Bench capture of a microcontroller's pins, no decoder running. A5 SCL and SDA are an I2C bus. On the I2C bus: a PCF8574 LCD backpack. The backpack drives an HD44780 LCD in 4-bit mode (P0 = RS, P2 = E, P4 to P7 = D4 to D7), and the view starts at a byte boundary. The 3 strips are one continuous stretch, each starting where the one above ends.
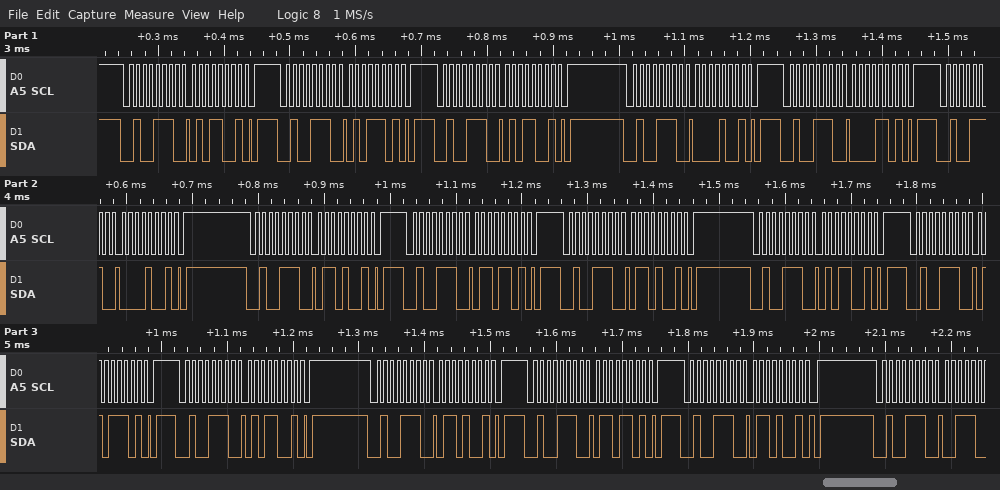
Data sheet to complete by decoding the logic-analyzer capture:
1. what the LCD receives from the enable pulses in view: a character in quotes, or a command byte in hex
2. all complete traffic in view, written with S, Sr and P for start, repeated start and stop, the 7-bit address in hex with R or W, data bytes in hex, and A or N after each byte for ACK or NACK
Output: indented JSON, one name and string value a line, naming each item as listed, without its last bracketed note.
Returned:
{
  "what the LCD receives from the enable pulses in view: a character in quotes, or a command byte in hex": "'P' 'e'",
  "all complete traffic in view, written with S, Sr and P for start, repeated start and stop, the 7-bit address in hex with R or W, data bytes in hex, and A or N after each byte for ACK or NACK": "S 27W A 59 A P S 27W A 5D A P S 27W A 59 A P S 27W A 09 A P S 27W A 0D A P S 27W A 09 A P S 27W A 69 A P S 27W A 6D A P S 27W A 69 A P S 27W A 59 A P S 27W A 5D A P S 27W A 59 A P S 27W A 69 A P S 27W A 6D A P S 27W A 69 A P S 27W A"
}
